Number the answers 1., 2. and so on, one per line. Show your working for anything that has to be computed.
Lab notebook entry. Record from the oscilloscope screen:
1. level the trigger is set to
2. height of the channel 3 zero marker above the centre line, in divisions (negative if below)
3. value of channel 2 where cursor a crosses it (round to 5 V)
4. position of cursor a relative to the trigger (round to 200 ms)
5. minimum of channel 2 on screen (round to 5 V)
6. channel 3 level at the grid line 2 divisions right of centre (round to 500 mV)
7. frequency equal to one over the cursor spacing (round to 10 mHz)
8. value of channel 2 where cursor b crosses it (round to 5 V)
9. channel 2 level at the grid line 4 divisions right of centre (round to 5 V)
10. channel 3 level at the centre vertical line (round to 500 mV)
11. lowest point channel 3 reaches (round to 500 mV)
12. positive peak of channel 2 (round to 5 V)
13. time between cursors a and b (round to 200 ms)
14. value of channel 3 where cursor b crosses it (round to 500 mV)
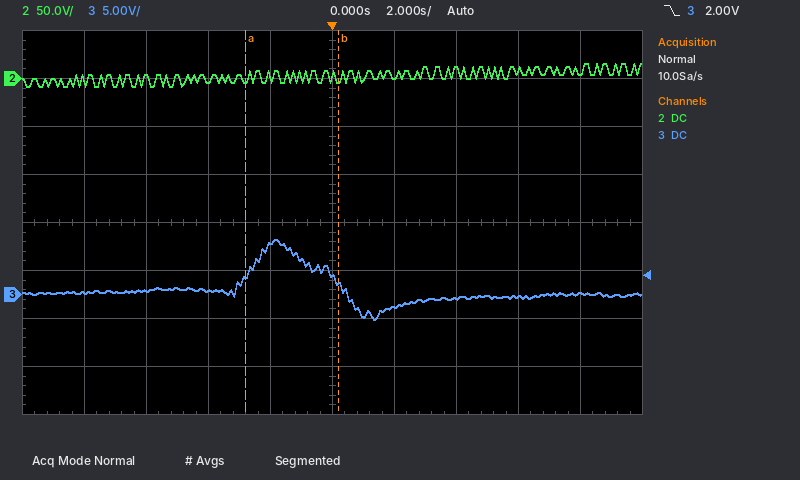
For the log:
1. 2.00 V
2. -1.5 div
3. 0 V
4. -2.8 s
5. -10 V
6. -500 mV
7. 1 / 3.0 s ≈ 330 mHz
8. 0 V
9. 5 V
10. 2.0 V
11. -2.5 V
12. 15 V
13. 3.0 s
14. 1.0 V
